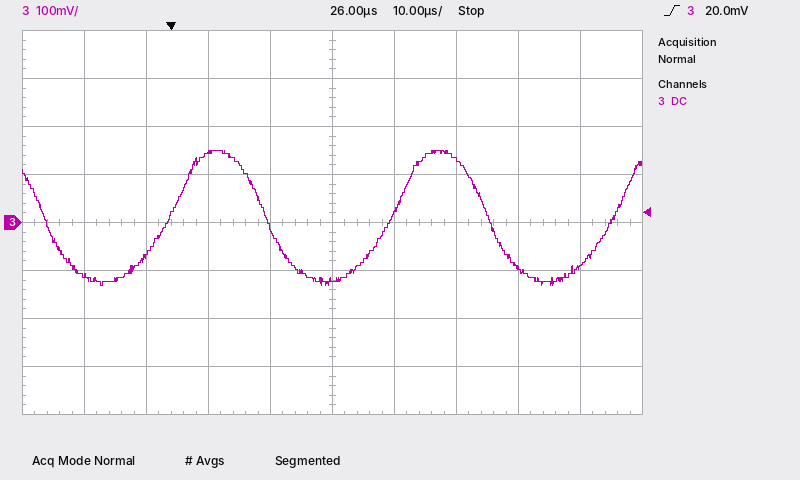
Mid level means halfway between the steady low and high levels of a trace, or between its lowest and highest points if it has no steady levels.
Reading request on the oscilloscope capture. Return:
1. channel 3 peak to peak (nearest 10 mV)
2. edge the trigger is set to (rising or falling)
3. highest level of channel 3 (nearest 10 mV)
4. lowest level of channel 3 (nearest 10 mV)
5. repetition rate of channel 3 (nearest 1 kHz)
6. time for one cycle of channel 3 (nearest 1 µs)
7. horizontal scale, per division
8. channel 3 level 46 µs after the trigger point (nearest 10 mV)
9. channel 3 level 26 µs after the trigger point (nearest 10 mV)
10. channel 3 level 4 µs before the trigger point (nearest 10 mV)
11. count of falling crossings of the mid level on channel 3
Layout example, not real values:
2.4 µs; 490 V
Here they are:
280 mV; rising; 150 mV; -130 mV; 28 kHz; 36 µs; 10 µs; 130 mV; -120 mV; -70 mV; 3
